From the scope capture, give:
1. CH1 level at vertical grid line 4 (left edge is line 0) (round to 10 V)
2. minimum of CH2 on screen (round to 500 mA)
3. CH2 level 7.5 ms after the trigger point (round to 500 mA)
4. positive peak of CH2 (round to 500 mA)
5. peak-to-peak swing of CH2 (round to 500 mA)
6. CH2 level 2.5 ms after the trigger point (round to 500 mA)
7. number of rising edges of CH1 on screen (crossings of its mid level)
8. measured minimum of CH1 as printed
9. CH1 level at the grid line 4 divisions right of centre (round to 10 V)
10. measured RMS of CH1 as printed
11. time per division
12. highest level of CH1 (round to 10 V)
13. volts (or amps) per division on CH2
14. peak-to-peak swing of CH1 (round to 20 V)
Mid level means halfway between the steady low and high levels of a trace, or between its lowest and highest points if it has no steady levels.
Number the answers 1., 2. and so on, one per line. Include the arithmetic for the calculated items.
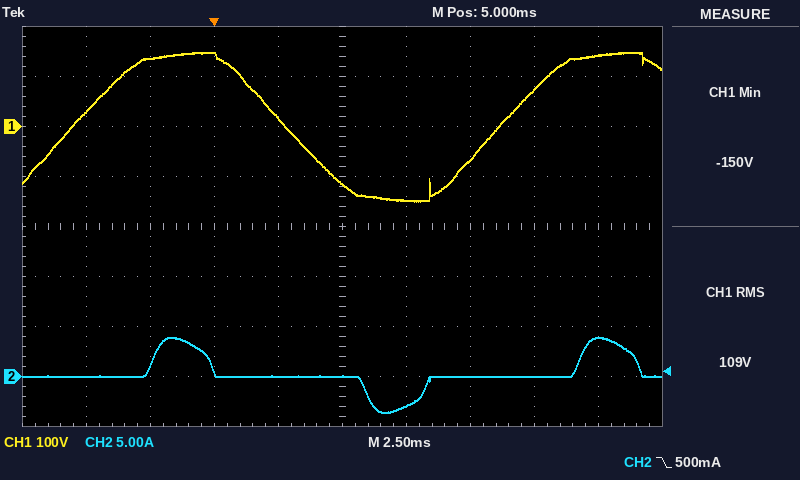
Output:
1. 20 V
2. -3.5 A
3. -3.0 A
4. 4.0 A
5. 4.0 A − (-3.5 A) = 7.5 A
6. 0.0 A
7. 2
8. -150 V
9. 140 V
10. 109 V
11. 2.5 ms
12. 150 V
13. 5 A
14. 300 V
